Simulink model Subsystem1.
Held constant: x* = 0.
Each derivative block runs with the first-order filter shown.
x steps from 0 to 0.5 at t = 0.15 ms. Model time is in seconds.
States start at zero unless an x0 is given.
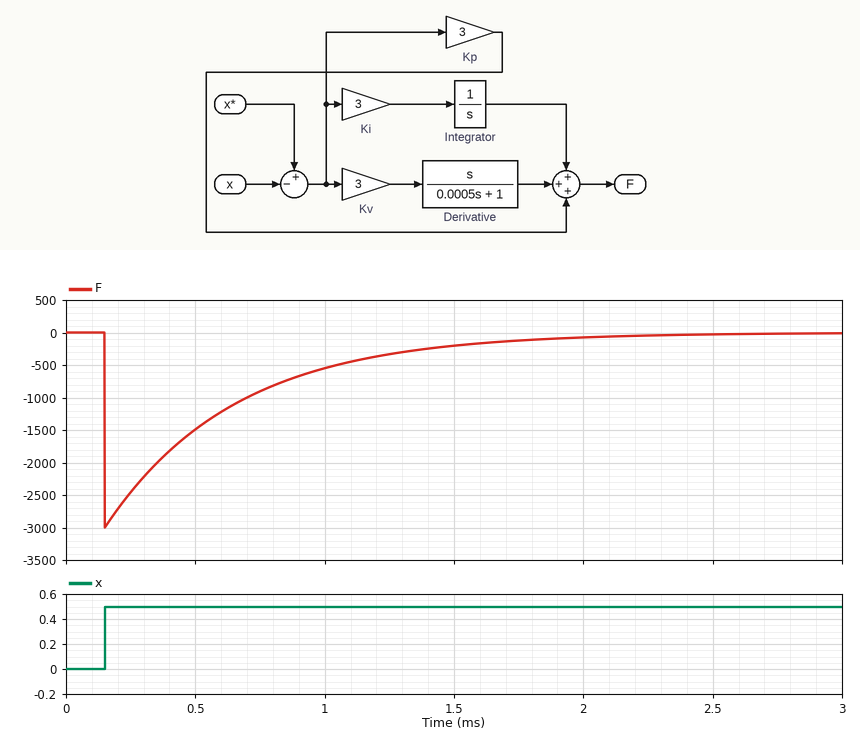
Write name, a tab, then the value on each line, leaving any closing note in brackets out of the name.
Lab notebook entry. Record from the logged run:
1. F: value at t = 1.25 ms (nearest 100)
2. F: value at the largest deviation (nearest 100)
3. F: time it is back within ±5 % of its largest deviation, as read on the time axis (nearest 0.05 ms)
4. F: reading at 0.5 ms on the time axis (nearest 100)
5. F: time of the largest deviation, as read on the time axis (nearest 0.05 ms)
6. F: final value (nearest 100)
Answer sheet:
F: value at t = 1.25 ms	-300
F: value at the largest deviation	-3000
F: time it is back within ±5 % of its largest deviation, as read on the time axis	1.65 ms
F: reading at 0.5 ms on the time axis	-1500
F: time of the largest deviation, as read on the time axis	0.15 ms
F: final value	0
